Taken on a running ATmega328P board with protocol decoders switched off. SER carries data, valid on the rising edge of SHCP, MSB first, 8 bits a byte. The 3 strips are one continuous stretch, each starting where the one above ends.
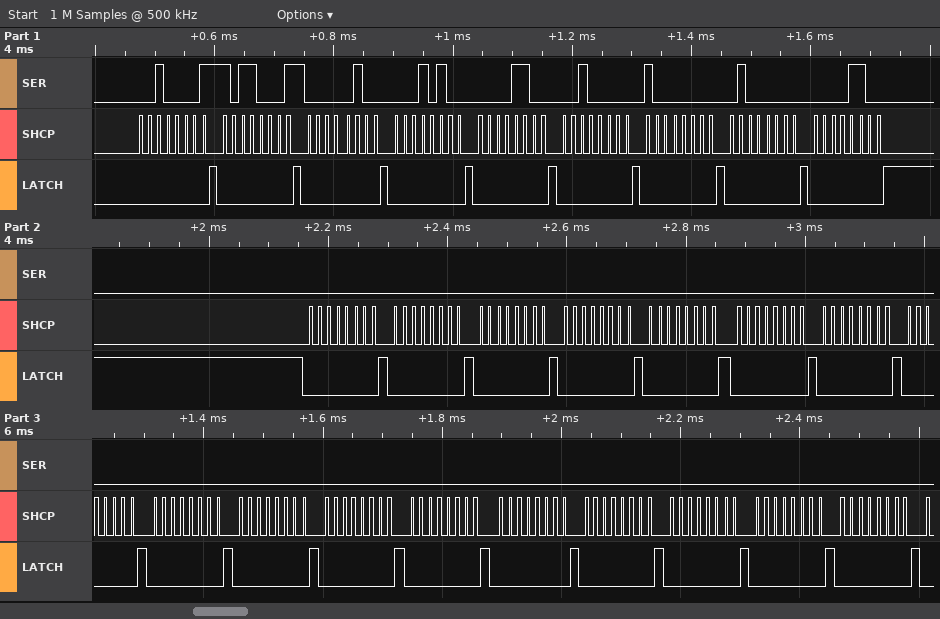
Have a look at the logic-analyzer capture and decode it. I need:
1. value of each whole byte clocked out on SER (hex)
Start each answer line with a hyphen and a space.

- 21 B1 04 14 0C 20 80 40 0C 00 00 00 00 00 00 00 00 00 00 00 00 00 00 00 00 00
